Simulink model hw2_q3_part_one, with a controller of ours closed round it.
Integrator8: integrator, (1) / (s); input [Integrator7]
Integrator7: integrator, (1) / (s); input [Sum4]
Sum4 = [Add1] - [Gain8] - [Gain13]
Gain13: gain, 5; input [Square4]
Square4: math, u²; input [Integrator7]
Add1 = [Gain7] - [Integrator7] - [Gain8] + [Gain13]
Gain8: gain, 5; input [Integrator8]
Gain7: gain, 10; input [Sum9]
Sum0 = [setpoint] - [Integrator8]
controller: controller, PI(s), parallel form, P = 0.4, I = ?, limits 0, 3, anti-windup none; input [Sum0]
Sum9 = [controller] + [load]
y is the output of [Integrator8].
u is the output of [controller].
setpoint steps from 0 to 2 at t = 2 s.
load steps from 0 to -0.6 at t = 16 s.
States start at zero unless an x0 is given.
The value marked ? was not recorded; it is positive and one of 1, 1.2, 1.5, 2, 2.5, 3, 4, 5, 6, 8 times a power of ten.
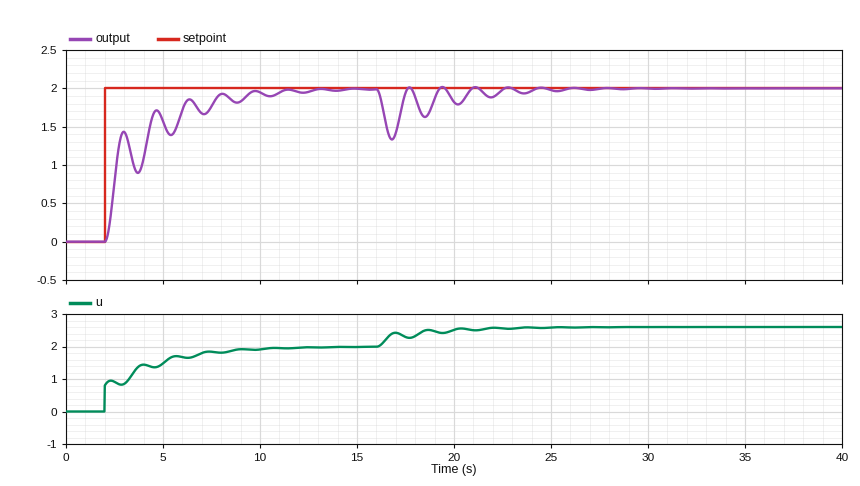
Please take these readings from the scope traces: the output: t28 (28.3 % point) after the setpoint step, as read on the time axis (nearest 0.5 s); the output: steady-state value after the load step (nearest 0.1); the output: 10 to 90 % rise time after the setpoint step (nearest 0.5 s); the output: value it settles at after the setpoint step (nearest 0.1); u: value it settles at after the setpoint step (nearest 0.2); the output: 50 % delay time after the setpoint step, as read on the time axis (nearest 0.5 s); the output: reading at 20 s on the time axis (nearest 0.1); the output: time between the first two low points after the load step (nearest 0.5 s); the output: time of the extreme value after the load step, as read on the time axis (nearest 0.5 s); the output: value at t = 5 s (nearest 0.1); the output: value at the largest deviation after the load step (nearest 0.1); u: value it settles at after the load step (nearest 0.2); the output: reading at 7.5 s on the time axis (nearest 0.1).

2.5 s
2.0
4.0 s
2.0
2.0
2.5 s
1.8
1.5 s
17.0 s
1.6
1.3
2.6
1.8
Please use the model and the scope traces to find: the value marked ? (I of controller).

0.5
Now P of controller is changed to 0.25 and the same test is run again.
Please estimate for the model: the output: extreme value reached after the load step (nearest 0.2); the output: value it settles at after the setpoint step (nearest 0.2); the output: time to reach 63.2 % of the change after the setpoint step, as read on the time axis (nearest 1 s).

1.2
2.0
3 s
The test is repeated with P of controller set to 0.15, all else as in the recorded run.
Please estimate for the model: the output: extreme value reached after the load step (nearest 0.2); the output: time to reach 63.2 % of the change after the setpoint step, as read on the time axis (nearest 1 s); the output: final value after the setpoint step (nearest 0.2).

1.2
4 s
2.0
